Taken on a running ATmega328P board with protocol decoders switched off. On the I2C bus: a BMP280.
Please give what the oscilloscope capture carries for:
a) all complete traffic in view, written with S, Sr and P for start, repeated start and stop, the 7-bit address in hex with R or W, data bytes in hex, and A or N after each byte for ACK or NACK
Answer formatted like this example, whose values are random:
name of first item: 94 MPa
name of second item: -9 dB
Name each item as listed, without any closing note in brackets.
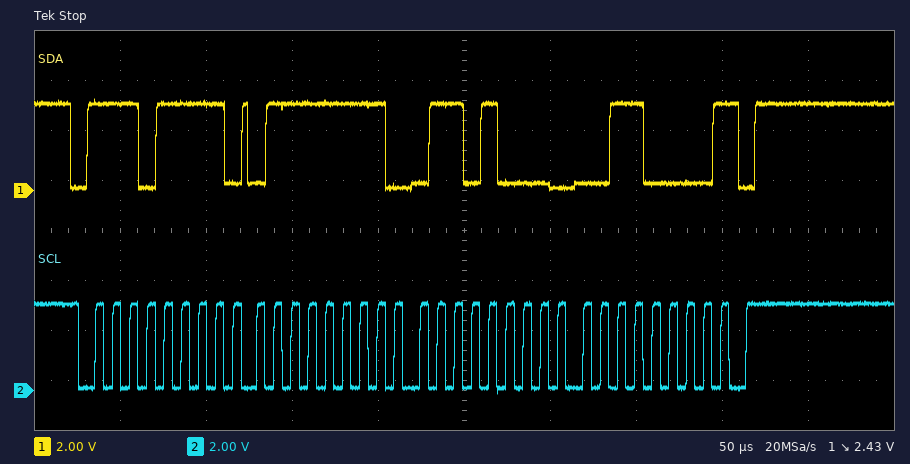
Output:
all complete traffic in view, written with S, Sr and P for start, repeated start and stop, the 7-bit address in hex with R or W, data bytes in hex, and A or N after each byte for ACK or NACK: S 77R A 7F A 68 A 30 N P
